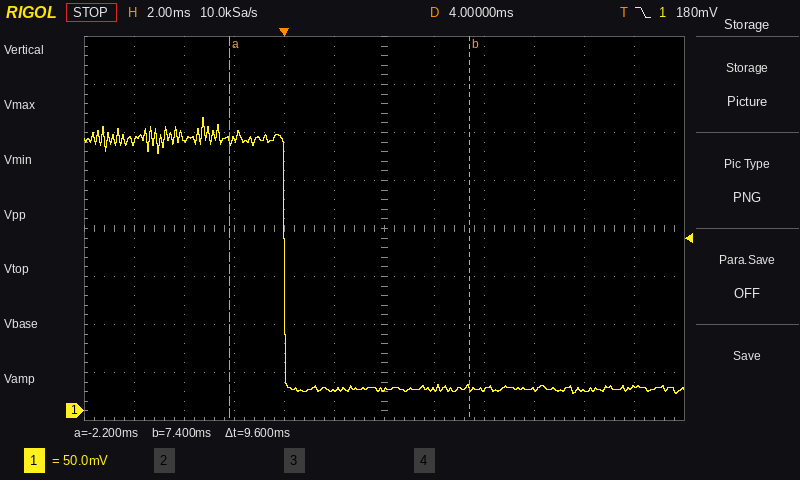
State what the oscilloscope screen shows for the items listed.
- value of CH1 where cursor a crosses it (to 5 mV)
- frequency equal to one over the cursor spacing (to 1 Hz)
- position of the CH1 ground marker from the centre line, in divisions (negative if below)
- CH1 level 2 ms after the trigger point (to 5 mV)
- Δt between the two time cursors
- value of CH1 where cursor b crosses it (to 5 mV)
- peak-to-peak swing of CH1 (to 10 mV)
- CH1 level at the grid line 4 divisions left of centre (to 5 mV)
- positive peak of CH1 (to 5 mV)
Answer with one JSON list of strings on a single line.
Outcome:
["280 mV", "104 Hz", "-3.8 div", "20 mV", "9.6 ms", "25 mV", "290 mV", "285 mV", "305 mV"]
